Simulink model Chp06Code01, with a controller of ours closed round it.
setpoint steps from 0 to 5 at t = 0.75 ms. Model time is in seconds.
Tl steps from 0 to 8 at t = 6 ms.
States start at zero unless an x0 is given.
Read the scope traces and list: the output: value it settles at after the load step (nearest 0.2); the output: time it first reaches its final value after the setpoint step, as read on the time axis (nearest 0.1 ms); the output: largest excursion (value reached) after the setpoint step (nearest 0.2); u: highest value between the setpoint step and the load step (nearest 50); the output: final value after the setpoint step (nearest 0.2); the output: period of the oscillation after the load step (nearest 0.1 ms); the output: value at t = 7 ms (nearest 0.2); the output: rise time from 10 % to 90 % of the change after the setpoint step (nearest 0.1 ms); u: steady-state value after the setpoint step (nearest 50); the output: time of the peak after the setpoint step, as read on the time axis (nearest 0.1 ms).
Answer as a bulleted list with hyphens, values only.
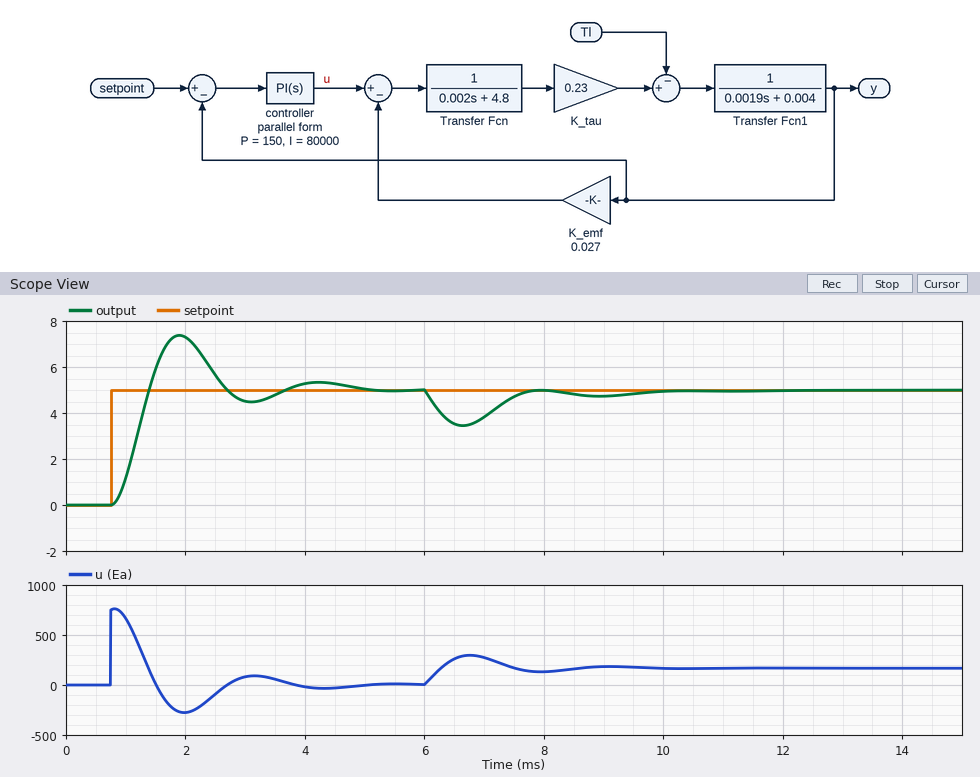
- 5.0
- 1.4 ms
- 7.4
- 750
- 5.0
- 2.3 ms
- 3.8
- 0.4 ms
- 0
- 1.9 ms
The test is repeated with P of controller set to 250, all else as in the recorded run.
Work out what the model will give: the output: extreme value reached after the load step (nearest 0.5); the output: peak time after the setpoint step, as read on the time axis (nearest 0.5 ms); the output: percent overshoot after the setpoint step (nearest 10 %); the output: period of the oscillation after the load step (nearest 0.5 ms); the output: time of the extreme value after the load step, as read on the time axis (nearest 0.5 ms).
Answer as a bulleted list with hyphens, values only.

- 4.0
- 1.5 ms
- 50 %
- 1.5 ms
- 6.5 ms
